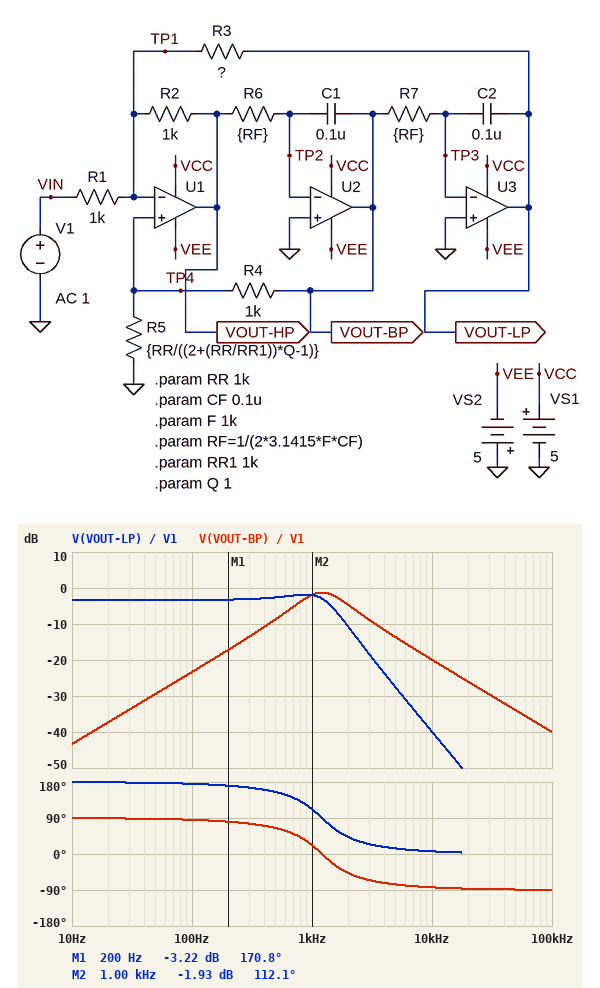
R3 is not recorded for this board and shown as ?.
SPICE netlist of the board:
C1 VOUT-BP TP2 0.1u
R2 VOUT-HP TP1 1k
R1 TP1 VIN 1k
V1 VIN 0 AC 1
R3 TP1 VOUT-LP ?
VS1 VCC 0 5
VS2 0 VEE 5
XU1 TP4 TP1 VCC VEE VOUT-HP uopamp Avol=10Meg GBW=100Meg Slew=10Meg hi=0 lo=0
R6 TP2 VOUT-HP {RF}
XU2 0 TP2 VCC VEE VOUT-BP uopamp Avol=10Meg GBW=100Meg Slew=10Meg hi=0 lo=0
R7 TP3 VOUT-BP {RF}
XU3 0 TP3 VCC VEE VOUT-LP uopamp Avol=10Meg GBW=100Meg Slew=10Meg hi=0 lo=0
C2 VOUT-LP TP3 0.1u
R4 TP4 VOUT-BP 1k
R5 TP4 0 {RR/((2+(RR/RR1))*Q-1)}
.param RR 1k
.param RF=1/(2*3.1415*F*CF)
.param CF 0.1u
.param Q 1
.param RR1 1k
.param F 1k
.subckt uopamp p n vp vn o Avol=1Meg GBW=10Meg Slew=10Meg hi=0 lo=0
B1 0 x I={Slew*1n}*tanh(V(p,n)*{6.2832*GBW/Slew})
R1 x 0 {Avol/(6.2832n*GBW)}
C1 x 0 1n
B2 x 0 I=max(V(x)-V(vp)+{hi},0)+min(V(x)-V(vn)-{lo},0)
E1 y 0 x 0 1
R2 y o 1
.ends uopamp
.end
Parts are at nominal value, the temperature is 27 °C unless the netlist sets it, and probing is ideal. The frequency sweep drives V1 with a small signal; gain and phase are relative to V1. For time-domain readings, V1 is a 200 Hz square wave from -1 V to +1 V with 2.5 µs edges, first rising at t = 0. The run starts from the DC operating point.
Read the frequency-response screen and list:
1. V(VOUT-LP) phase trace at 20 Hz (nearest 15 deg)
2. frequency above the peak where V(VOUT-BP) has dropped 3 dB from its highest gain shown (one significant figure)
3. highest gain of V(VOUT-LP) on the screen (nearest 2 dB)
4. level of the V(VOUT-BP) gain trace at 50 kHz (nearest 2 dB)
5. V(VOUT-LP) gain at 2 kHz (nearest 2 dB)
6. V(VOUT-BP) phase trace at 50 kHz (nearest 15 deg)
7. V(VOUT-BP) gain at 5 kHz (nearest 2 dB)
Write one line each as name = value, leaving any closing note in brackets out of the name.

V(VOUT-LP) phase trace at 20 Hz = 180 deg
frequency above the peak where V(VOUT-BP) has dropped 3 dB from its highest gain shown = 2 kHz
highest gain of V(VOUT-LP) on the screen = -2 dB
level of the V(VOUT-BP) gain trace at 50 kHz = -34 dB
V(VOUT-LP) gain at 2 kHz = -10 dB
V(VOUT-BP) phase trace at 50 kHz = -90 deg
V(VOUT-BP) gain at 5 kHz = -14 dB
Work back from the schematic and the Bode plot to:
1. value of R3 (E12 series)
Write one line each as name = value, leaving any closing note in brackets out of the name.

value of R3 = 680 Ω
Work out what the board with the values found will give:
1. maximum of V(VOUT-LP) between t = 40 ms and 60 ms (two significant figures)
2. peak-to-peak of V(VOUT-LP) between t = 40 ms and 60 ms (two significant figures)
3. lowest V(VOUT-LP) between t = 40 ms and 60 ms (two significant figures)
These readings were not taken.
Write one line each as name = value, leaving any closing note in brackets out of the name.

maximum of V(VOUT-LP) between t = 40 ms and 60 ms = 930 mV
peak-to-peak of V(VOUT-LP) between t = 40 ms and 60 ms = 1.9 V
lowest V(VOUT-LP) between t = 40 ms and 60 ms = -930 mV
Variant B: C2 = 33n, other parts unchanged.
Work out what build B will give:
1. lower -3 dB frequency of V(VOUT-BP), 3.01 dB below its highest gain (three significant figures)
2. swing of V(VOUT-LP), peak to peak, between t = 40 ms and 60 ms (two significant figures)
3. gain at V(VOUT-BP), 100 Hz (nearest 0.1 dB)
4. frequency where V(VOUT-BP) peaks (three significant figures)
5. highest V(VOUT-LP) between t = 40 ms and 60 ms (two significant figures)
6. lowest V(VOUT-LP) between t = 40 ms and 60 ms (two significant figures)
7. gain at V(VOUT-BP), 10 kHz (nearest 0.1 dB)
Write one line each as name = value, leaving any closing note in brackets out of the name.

lower -3 dB frequency of V(VOUT-BP), 3.01 dB below its highest gain = 1.61 kHz
swing of V(VOUT-LP), peak to peak, between t = 40 ms and 60 ms = 2.5 V
gain at V(VOUT-BP), 100 Hz = -33.0 dB
frequency where V(VOUT-BP) peaks = 2.11 kHz
highest V(VOUT-LP) between t = 40 ms and 60 ms = 1.2 V
lowest V(VOUT-LP) between t = 40 ms and 60 ms = -1.2 V
gain at V(VOUT-BP), 10 kHz = -19.7 dB
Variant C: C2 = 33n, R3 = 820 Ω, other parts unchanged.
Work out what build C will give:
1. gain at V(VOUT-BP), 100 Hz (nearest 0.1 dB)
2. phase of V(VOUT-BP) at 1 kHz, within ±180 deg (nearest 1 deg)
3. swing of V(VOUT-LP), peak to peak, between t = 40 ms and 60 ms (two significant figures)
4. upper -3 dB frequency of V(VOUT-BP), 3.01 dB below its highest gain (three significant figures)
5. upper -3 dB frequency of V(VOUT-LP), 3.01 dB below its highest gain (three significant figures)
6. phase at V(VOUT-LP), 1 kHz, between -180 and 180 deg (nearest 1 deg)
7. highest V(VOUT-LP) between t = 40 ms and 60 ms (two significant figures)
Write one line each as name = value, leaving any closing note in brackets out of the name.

gain at V(VOUT-BP), 100 Hz = -31.3 dB
phase of V(VOUT-BP) at 1 kHz, within ±180 deg = 68 deg
swing of V(VOUT-LP), peak to peak, between t = 40 ms and 60 ms = 3.0 V
upper -3 dB frequency of V(VOUT-BP), 3.01 dB below its highest gain = 2.53 kHz
upper -3 dB frequency of V(VOUT-LP), 3.01 dB below its highest gain = 2.26 kHz
phase at V(VOUT-LP), 1 kHz, between -180 and 180 deg = 158 deg
highest V(VOUT-LP) between t = 40 ms and 60 ms = 1.5 V
